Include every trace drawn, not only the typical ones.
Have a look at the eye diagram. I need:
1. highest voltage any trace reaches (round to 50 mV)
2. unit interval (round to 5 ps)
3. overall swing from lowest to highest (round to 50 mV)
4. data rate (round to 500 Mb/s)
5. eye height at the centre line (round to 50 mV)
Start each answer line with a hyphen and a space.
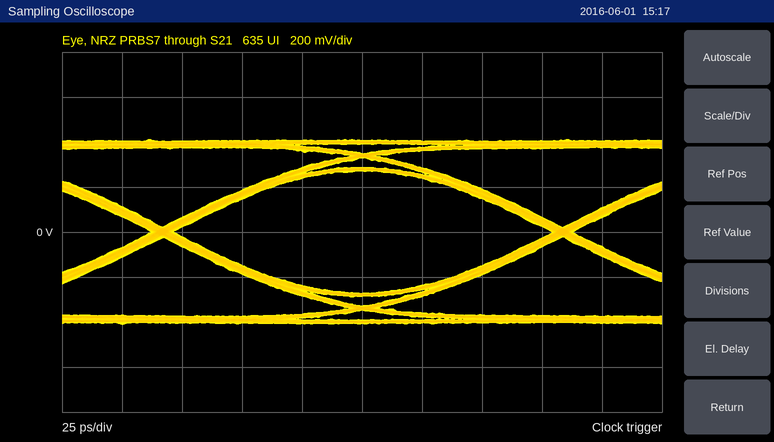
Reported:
- 400 mV
- 165 ps
- 800 mV
- 6.0 Gb/s
- 550 mV
